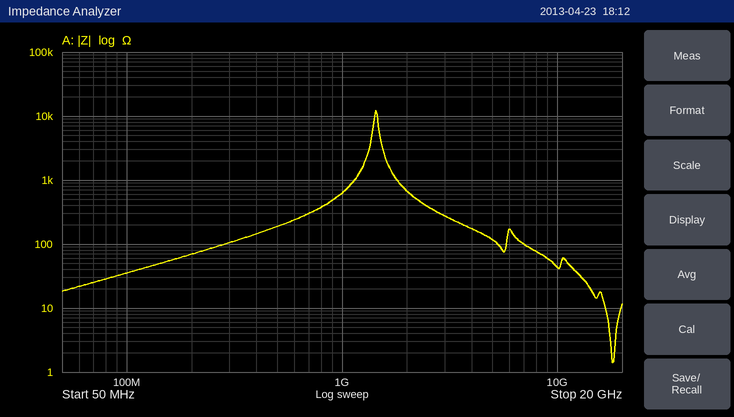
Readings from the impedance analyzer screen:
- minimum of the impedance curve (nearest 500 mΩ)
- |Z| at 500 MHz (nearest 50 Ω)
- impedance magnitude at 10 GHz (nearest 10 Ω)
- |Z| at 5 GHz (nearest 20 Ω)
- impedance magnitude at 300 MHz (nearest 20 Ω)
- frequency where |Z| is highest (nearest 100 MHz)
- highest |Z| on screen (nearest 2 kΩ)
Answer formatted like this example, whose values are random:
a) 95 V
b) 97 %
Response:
a) 1.5 Ω
b) 200 Ω
c) 40 Ω
d) 120 Ω
e) 100 Ω
f) 1.4 GHz
g) 12 kΩ
